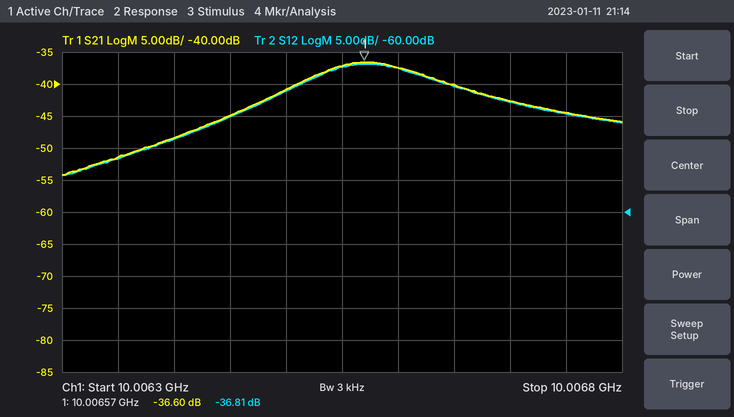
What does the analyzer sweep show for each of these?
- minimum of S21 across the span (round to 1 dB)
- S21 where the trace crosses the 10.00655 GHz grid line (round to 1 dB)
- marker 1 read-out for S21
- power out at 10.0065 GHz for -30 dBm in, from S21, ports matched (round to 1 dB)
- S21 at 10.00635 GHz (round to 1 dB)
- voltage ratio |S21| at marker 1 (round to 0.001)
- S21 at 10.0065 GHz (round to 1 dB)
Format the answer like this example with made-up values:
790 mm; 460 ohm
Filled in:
-54 dB; -37 dB; -36.60 dB; -71 dBm; -51 dB; 0.015; -41 dB
